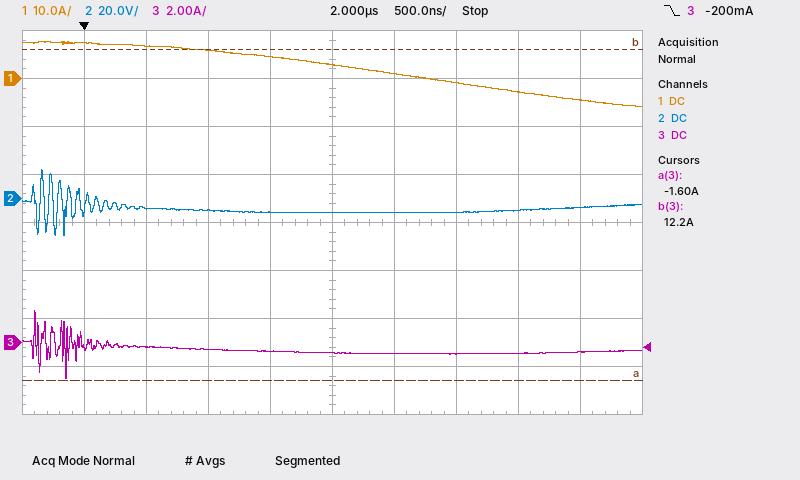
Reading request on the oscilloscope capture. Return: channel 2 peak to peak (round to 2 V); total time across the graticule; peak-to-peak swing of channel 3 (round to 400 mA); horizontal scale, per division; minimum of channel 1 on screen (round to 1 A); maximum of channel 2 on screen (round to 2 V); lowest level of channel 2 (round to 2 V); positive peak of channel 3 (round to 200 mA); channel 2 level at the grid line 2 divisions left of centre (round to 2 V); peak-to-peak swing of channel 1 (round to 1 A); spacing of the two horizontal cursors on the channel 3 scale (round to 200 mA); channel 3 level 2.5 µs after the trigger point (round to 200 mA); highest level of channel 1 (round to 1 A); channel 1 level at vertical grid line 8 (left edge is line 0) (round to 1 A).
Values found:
28 V
5 µs
2.8 A
500 ns
-6 A
12 V
-16 V
1.4 A
-4 V
14 A
13.8 A
-400 mA
8 A
-3 A
